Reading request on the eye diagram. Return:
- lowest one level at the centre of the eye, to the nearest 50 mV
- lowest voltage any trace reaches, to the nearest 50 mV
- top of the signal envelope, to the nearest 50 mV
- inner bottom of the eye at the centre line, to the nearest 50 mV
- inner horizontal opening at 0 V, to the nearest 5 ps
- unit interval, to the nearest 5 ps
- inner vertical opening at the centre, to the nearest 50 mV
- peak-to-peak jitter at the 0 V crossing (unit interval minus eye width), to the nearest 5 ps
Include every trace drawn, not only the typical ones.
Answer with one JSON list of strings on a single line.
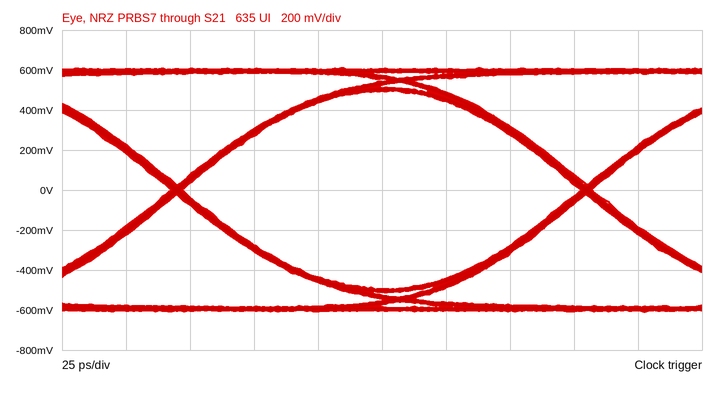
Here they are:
["500 mV", "-600 mV", "600 mV", "-500 mV", "155 ps", "160 ps", "1.00 V", "5 ps"]
